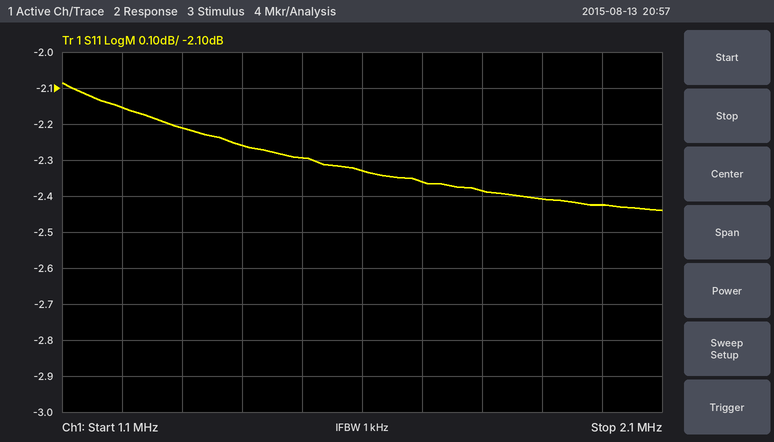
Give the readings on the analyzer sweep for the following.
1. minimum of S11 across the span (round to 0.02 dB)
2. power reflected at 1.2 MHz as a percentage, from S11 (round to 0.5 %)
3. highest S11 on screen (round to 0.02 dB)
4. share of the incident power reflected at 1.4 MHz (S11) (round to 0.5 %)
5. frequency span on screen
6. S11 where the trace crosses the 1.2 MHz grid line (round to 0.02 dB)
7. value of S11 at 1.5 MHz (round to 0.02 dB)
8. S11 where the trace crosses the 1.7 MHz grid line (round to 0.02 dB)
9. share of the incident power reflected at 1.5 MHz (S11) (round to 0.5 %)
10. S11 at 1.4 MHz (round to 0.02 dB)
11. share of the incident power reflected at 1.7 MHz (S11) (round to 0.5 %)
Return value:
-2.44 dB
61.0 %
-2.08 dB
59.5 %
1 MHz
-2.16 dB
-2.30 dB
-2.36 dB
59.0 %
-2.26 dB
58.0 %
